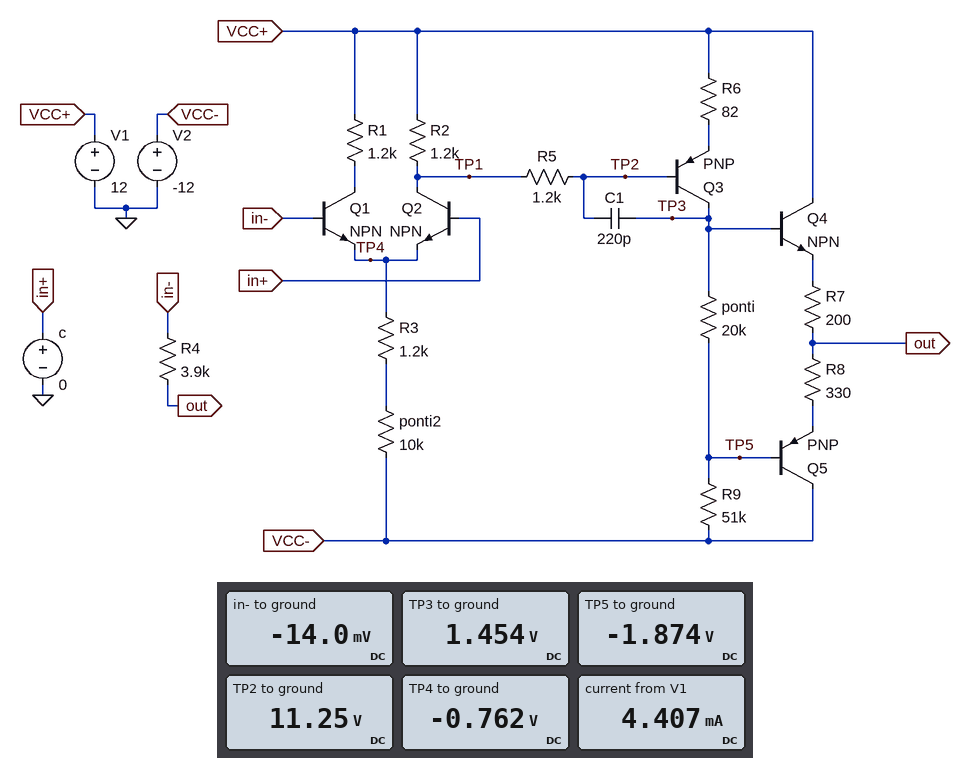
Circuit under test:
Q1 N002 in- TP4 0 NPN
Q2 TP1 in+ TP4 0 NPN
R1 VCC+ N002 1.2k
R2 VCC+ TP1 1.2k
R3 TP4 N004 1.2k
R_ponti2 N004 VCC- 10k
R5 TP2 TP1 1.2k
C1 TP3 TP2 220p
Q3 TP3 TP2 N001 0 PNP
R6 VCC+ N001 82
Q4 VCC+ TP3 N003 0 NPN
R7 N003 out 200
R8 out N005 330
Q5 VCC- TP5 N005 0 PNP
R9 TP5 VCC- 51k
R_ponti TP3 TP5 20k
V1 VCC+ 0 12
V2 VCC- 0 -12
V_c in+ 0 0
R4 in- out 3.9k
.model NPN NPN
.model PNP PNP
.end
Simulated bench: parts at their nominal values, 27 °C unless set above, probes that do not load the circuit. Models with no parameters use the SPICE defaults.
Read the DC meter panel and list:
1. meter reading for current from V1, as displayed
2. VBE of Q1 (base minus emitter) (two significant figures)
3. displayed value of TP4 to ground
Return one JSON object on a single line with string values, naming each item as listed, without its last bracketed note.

{"meter reading for current from V1, as displayed": "4.407 mA", "VBE of Q1 (base minus emitter)": "750 mV", "displayed value of TP4 to ground": "-0.762 V"}
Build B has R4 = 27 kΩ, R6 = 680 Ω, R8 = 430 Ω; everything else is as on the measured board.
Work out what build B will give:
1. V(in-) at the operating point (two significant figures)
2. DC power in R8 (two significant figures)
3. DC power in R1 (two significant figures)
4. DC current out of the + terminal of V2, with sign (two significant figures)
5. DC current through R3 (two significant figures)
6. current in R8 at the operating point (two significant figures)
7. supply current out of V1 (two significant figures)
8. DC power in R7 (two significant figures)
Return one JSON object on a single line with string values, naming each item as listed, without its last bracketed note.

{"V(in-) at the operating point": "-26 mV", "DC power in R8": "3.4 mW", "DC power in R1": "85 µW", "DC current out of the + terminal of V2, with sign": "-4.0 mA", "DC current through R3": "1.0 mA", "current in R8 at the operating point": "2.8 mA", "supply current out of V1": "4.0 mA", "DC power in R7": "1.6 mW"}
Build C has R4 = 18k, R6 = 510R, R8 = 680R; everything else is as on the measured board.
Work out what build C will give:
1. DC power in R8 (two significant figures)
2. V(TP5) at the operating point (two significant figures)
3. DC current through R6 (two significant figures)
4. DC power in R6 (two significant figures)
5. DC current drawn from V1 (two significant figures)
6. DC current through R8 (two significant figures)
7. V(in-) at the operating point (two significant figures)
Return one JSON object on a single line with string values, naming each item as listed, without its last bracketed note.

{"DC power in R8": "3.0 mW", "V(TP5) at the operating point": "-2.2 V", "DC current through R6": "190 µA", "DC power in R6": "19 µW", "DC current drawn from V1": "3.3 mA", "DC current through R8": "2.1 mA", "V(in-) at the operating point": "-22 mV"}
